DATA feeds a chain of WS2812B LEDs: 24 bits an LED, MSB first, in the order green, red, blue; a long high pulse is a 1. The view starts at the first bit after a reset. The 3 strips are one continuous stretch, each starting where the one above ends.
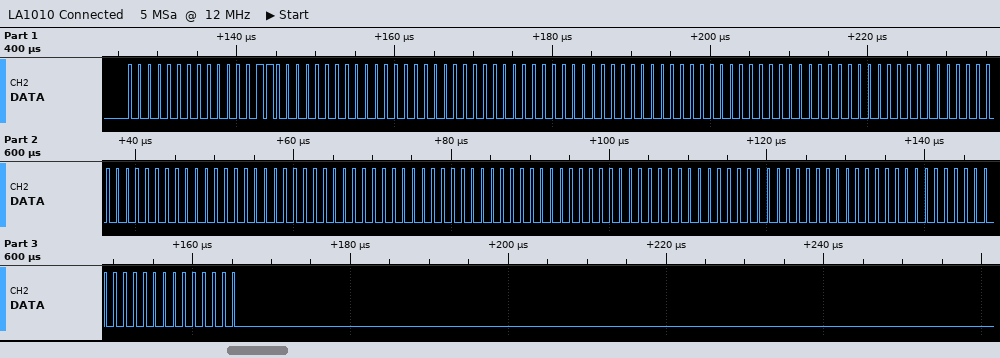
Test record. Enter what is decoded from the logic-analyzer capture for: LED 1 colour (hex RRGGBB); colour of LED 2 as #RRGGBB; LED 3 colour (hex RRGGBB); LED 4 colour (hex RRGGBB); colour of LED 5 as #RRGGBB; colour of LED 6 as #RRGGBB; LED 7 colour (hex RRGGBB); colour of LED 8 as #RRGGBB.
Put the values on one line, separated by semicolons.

#060000; #000000; #000000; #000000; #000000; #000000; #000000; #000000
